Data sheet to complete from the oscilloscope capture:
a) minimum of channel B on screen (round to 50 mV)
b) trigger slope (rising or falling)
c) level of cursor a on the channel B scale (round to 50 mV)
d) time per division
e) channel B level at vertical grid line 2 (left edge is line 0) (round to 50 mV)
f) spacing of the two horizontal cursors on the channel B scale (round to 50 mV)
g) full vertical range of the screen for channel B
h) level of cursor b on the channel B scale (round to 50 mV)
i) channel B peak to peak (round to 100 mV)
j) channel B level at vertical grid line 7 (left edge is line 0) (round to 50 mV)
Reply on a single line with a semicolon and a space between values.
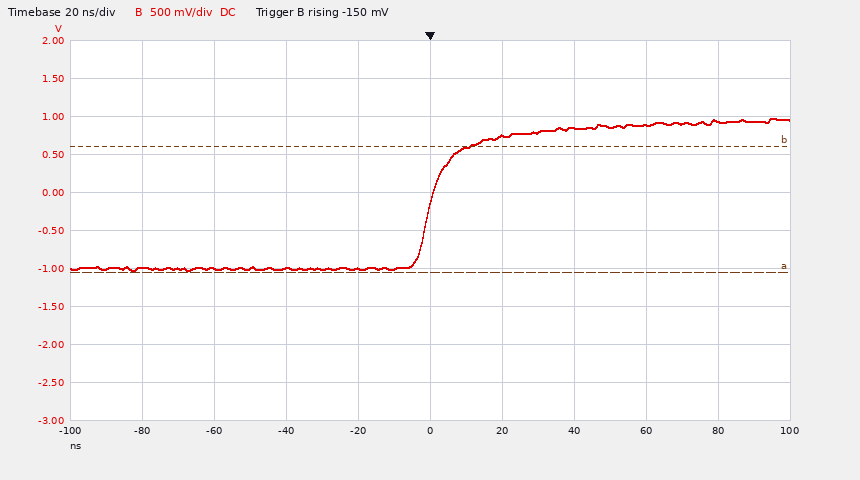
-1.05 V; rising; -1.05 V; 20 ns; -1.00 V; 1.65 V; 5 V; 600 mV; 2.00 V; 850 mV
